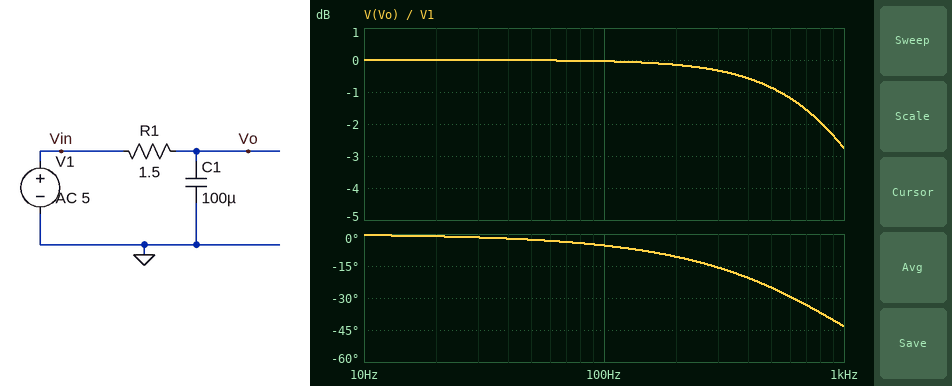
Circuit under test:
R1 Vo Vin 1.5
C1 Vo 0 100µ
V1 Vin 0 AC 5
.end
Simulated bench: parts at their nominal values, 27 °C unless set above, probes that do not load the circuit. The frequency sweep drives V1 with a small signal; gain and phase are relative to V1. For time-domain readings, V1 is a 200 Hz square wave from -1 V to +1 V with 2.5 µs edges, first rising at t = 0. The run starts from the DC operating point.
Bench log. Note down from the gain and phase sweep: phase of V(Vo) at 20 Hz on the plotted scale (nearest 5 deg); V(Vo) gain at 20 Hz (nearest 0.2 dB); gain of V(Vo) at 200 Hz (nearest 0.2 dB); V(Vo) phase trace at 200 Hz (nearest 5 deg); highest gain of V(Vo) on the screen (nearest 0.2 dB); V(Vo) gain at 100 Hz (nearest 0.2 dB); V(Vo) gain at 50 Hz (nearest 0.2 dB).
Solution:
0 deg
0 dB
-0.2 dB
-10 deg
0 dB
0 dB
0 dB
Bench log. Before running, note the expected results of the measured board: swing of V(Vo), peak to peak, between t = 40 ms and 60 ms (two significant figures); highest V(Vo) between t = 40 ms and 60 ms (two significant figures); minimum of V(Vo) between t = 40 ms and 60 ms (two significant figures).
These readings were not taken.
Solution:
2.0 V
1.0 V
-1.0 V
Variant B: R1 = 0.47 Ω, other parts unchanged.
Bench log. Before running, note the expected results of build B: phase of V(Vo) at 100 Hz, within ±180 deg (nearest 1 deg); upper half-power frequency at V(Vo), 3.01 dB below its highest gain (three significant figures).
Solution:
-2 deg
3.39 kHz
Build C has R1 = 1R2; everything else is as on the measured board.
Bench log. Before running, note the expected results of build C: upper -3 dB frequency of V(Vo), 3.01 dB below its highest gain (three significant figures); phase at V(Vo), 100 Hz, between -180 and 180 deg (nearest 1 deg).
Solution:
1.33 kHz
-4 deg
